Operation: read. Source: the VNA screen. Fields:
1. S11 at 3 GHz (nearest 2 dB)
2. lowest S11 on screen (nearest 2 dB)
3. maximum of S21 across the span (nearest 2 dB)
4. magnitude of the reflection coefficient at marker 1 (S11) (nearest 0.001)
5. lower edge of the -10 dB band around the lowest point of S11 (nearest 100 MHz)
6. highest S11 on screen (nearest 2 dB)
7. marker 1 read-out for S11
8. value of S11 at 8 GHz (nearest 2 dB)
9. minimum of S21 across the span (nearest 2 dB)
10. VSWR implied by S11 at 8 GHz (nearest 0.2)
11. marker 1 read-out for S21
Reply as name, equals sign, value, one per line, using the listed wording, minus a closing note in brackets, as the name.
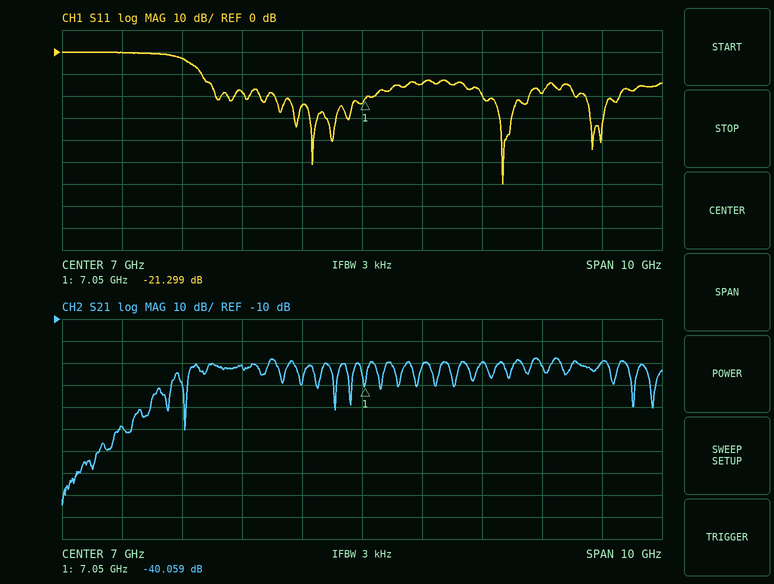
S11 at 3 GHz = 0 dB
lowest S11 on screen = -60 dB
maximum of S21 across the span = -28 dB
magnitude of the reflection coefficient at marker 1 (S11) = 0.086
lower edge of the -10 dB band around the lowest point of S11 = 4.3 GHz
highest S11 on screen = 0 dB
marker 1 read-out for S11 = -21.299 dB
value of S11 at 8 GHz = -14 dB
minimum of S21 across the span = -94 dB
VSWR implied by S11 at 8 GHz = 1.4
marker 1 read-out for S21 = -40.059 dB
